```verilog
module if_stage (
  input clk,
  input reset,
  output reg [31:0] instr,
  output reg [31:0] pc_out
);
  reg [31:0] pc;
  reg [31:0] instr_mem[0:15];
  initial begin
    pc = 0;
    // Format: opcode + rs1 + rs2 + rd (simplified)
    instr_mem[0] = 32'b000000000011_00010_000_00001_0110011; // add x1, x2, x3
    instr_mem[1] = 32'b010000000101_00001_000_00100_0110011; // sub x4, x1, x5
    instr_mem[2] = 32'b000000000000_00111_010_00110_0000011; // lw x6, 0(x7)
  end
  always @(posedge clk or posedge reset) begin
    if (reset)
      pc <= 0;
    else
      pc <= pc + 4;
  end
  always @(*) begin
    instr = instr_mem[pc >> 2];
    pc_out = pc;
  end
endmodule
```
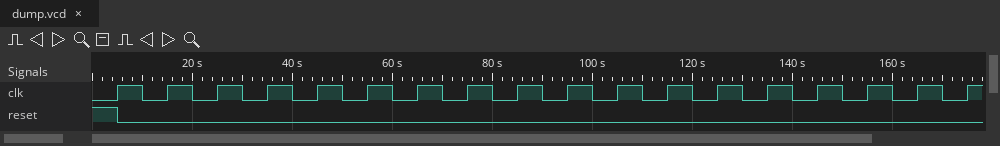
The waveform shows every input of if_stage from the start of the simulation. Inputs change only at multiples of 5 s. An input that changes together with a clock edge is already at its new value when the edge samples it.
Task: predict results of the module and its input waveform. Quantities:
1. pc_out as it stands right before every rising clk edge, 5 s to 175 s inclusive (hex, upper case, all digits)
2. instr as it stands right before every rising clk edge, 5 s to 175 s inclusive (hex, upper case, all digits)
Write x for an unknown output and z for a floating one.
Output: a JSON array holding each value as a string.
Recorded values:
["00000000, 00000004, 00000008, 0000000C, 00000010, 00000014, 00000018, 0000001C, 00000020, 00000024, 00000028, 0000002C, 00000030, 00000034, 00000038, 0000003C, 00000040, 00000044", "003100B3, 40508233, 0003A303, x, x, x, x, x, x, x, x, x, x, x, x, x, x, x"]
